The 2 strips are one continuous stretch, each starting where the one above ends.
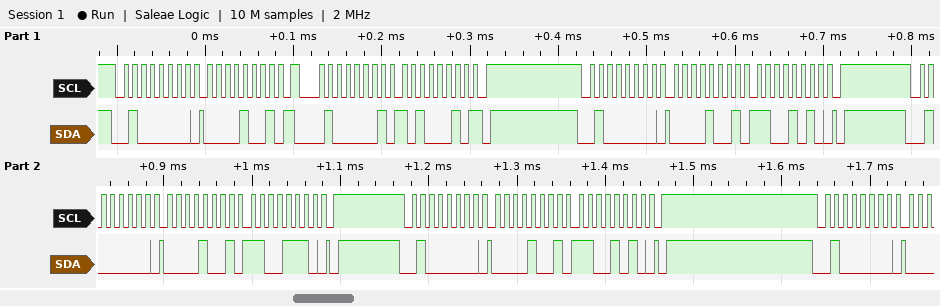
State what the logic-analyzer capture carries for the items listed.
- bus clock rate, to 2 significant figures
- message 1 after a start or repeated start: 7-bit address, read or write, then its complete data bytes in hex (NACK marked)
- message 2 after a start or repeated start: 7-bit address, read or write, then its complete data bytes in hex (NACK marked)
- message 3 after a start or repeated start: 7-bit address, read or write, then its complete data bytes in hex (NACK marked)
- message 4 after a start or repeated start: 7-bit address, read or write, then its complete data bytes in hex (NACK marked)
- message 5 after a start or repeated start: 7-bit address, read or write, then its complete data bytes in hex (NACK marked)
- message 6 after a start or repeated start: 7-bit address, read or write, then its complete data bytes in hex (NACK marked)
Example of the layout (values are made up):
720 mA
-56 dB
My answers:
100 kHz
0x20 write: 09
0x20 read: A2 NACK
0x20 write: 09 CA
0x20 write: 09 CE
0x20 write: 09 CA
0x20 write
